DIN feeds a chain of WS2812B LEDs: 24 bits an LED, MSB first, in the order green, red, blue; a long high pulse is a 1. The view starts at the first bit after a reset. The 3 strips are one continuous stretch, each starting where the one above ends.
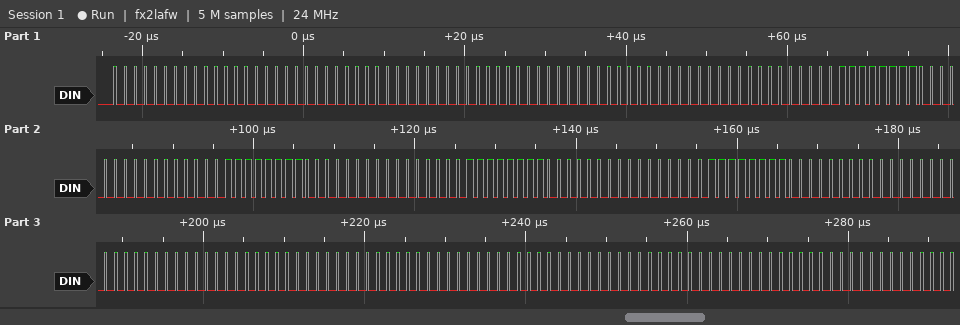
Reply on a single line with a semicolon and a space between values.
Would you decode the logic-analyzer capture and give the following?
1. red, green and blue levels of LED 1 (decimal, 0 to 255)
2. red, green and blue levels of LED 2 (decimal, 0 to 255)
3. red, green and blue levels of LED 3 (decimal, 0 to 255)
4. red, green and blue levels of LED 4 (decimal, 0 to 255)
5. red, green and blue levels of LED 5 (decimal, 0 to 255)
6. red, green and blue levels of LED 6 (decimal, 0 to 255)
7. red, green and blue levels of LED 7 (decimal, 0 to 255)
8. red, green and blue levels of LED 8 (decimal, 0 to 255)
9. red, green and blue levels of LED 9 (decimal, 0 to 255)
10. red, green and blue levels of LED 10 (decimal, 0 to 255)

0, 0, 0; 0, 0, 0; 0, 0, 0; 0, 255, 0; 0, 255, 0; 0, 255, 0; 0, 255, 0; 0, 0, 0; 0, 0, 0; 0, 0, 0
